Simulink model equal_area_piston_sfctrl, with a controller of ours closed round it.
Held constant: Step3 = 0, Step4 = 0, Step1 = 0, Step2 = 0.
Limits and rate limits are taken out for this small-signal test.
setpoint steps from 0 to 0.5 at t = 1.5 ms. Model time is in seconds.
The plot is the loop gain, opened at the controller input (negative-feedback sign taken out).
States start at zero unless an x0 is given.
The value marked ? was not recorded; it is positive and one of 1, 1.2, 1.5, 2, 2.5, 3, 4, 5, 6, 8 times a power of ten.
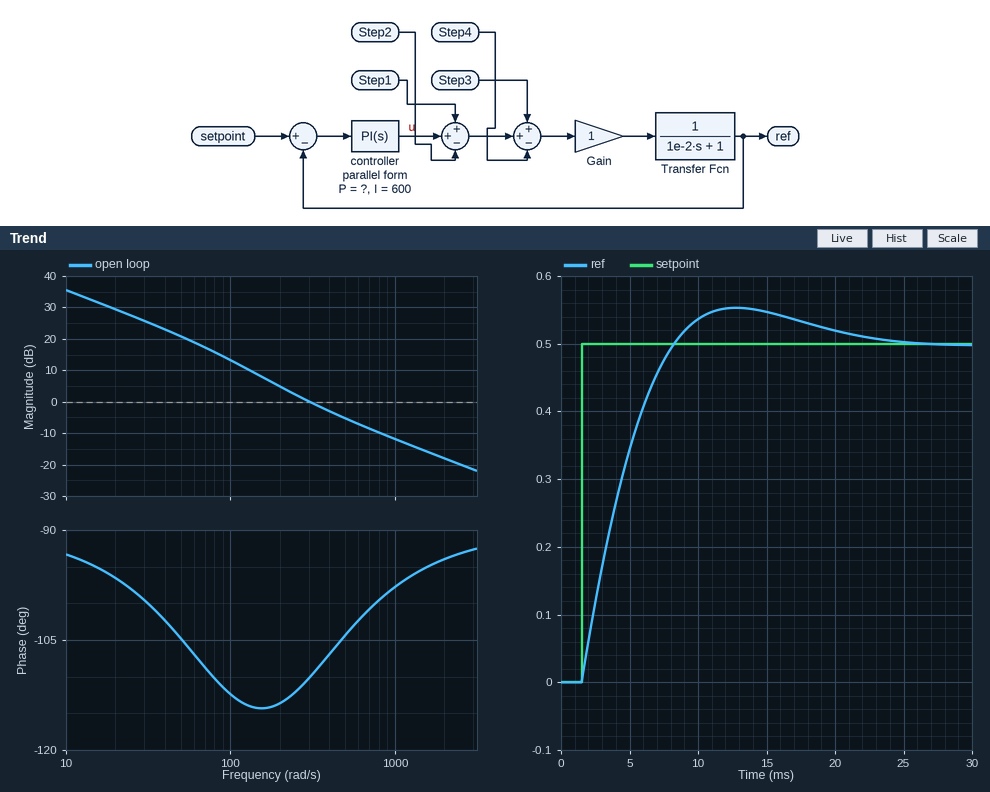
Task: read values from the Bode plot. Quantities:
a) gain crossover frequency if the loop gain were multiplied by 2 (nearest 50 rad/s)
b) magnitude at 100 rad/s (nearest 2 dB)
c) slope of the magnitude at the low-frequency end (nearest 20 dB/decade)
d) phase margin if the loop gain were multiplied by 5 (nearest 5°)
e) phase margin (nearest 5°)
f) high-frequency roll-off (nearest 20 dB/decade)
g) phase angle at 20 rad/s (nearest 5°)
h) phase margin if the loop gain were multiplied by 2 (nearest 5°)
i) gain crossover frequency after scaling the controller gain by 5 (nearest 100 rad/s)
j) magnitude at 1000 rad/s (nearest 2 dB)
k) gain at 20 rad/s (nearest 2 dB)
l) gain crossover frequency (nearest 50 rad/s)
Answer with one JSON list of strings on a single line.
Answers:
["550 rad/s", "14 dB", "-20 dB/decade", "85°", "70°", "-20 dB/decade", "-95°", "75°", "1300 rad/s", "-12 dB", "30 dB", "300 rad/s"]
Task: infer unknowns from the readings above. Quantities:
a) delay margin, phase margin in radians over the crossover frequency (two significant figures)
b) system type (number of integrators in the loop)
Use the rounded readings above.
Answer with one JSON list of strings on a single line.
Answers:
["0.0041 s", "1"]
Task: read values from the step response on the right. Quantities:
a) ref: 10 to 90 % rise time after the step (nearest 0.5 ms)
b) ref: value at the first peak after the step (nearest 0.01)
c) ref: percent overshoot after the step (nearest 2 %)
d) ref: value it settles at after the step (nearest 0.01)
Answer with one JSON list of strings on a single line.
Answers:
["5.0 ms", "0.55", "10 %", "0.50"]
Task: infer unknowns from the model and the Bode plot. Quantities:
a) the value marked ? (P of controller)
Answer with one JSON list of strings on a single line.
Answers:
["2.5"]
